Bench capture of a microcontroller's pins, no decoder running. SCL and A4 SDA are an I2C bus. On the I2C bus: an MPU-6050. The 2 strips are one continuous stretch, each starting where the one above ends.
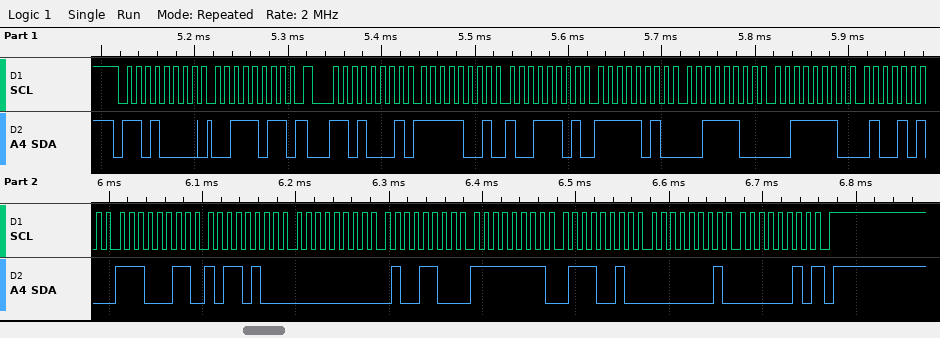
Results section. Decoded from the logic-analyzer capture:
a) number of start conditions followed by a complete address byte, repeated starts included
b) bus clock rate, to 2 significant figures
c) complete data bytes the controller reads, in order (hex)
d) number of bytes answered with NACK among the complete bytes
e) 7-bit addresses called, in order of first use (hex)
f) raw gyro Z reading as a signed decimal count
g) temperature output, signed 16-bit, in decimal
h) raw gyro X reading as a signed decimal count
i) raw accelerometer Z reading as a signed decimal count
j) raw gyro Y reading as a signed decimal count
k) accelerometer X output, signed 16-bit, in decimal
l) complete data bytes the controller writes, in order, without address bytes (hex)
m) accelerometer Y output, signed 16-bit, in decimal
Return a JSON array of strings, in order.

["2", "100 kHz", "F9 9D FA 3C 3E 4A E3 B4 00 4C FF 72 01 02", "1", "0x68", "258", "-7244", "76", "15946", "-142", "-1635", "3B", "-1476"]
